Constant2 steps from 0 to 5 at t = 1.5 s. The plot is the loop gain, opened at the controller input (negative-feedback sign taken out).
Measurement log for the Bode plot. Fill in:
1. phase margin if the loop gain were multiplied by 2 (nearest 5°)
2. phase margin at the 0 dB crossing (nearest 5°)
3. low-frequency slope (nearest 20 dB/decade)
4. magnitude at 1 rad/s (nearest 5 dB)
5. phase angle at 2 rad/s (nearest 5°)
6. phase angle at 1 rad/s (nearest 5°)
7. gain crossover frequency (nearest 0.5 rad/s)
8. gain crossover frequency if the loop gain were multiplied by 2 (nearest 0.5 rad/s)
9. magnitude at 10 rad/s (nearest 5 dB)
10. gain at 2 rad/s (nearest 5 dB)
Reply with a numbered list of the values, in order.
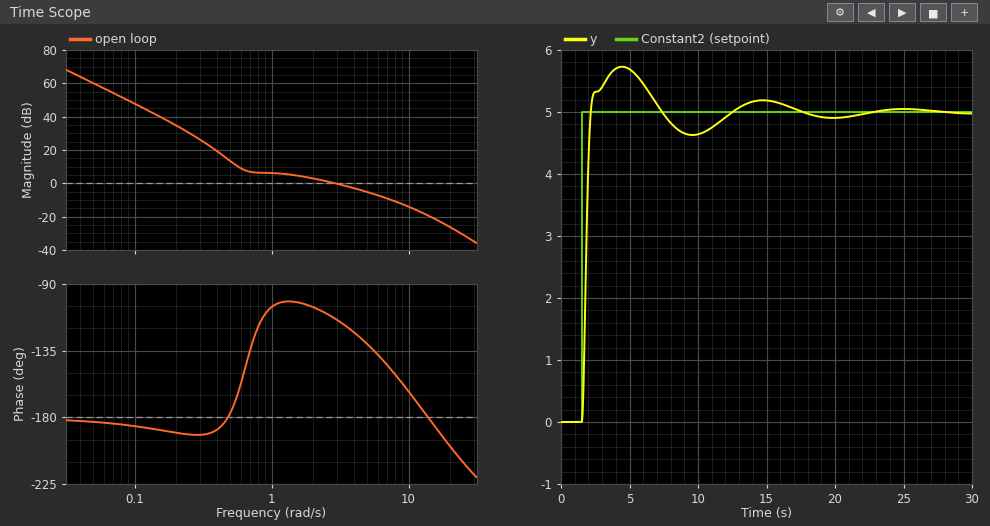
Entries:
1. 45°
2. 65°
3. -40 dB/decade
4. 5 dB
5. -105°
6. -105°
7. 3.0 rad/s
8. 5.5 rad/s
9. -15 dB
10. 5 dB
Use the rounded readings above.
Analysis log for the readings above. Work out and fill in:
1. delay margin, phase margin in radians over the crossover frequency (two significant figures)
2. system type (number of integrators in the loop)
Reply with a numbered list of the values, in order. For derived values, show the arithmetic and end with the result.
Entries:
1. 65 × π / 180 / 3 = 0.38 s
2. 2
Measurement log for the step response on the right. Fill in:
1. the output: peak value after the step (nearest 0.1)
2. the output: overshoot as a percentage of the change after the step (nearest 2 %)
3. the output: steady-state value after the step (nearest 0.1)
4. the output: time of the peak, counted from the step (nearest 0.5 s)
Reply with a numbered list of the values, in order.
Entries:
1. 5.7
2. 14 %
3. 5.0
4. 3.0 s
